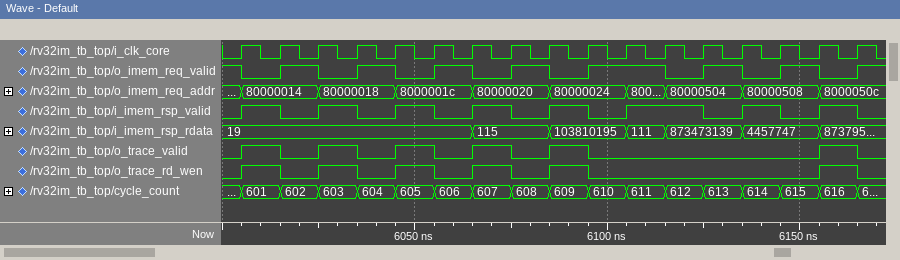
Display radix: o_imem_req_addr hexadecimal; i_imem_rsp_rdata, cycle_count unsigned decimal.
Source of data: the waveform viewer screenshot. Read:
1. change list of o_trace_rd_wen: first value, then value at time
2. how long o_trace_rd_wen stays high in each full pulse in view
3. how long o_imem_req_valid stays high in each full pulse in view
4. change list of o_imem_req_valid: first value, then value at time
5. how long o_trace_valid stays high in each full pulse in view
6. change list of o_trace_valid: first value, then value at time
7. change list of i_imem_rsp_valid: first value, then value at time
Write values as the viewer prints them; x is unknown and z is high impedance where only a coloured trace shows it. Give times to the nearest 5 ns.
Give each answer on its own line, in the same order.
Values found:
0, 1 at 6005 ns, 0 at 6015 ns, 1 at 6025 ns, 0 at 6035 ns, 1 at 6045 ns, 0 at 6055 ns, 1 at 6065 ns, 0 at 6075 ns, 1 at 6085 ns, 0 at 6095 ns, 1 at 6155 ns, 0 at 6165 ns
10 ns, 10 ns, 10 ns, 10 ns, 10 ns, 10 ns
10 ns, 10 ns, 10 ns, 10 ns, 20 ns, 10 ns, 10 ns
1, 0 at 6005 ns, 1 at 6015 ns, 0 at 6025 ns, 1 at 6035 ns, 0 at 6045 ns, 1 at 6055 ns, 0 at 6065 ns, 1 at 6075 ns, 0 at 6085 ns, 1 at 6095 ns, 0 at 6115 ns, 1 at 6125 ns, 0 at 6135 ns, 1 at 6145 ns, 0 at 6155 ns, 1 at 6165 ns
10 ns, 10 ns, 10 ns, 10 ns, 10 ns, 10 ns
0, 1 at 6005 ns, 0 at 6015 ns, 1 at 6025 ns, 0 at 6035 ns, 1 at 6045 ns, 0 at 6055 ns, 1 at 6065 ns, 0 at 6075 ns, 1 at 6085 ns, 0 at 6095 ns, 1 at 6155 ns, 0 at 6165 ns
0, 1 at 6005 ns, 0 at 6015 ns, 1 at 6025 ns, 0 at 6035 ns, 1 at 6045 ns, 0 at 6055 ns, 1 at 6065 ns, 0 at 6075 ns, 1 at 6085 ns, 0 at 6095 ns, 1 at 6105 ns, 0 at 6125 ns, 1 at 6135 ns, 0 at 6145 ns, 1 at 6155 ns, 0 at 6165 ns
